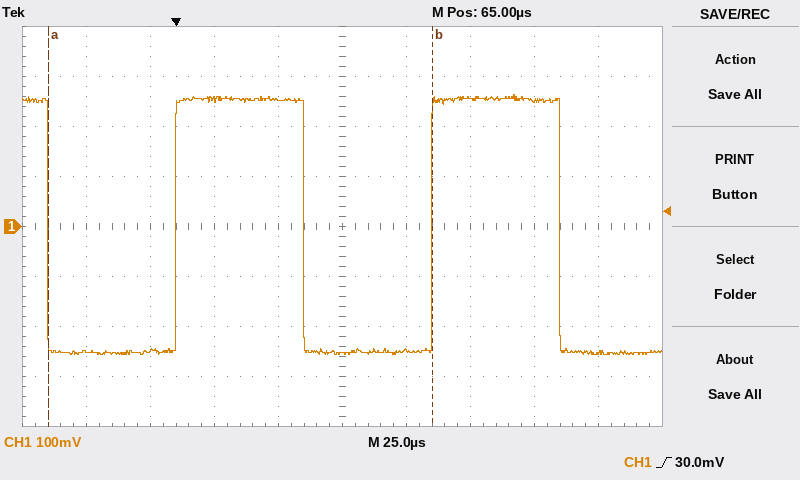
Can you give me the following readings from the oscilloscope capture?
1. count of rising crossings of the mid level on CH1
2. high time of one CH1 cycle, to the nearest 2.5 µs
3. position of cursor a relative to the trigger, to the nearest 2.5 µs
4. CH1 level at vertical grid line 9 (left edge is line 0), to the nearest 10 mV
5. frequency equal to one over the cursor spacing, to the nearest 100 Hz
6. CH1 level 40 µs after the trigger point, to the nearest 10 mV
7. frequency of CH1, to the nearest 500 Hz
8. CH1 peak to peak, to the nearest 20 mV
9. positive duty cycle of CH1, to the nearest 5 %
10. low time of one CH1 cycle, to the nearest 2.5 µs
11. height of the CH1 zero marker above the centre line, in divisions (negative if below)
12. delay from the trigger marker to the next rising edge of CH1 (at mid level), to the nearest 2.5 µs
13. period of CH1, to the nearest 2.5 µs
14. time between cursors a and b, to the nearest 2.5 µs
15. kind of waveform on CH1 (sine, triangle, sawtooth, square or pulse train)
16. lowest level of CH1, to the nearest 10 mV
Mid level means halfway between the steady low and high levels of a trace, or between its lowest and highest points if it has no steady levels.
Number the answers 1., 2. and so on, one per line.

1. 2
2. 50.0 µs
3. -50.0 µs
4. -250 mV
5. 6.7 kHz
6. 250 mV
7. 10.0 kHz
8. 520 mV
9. 50 %
10. 50.0 µs
11. 0.0 div
12. 100.0 µs
13. 100.0 µs
14. 150.0 µs
15. square
16. -260 mV
